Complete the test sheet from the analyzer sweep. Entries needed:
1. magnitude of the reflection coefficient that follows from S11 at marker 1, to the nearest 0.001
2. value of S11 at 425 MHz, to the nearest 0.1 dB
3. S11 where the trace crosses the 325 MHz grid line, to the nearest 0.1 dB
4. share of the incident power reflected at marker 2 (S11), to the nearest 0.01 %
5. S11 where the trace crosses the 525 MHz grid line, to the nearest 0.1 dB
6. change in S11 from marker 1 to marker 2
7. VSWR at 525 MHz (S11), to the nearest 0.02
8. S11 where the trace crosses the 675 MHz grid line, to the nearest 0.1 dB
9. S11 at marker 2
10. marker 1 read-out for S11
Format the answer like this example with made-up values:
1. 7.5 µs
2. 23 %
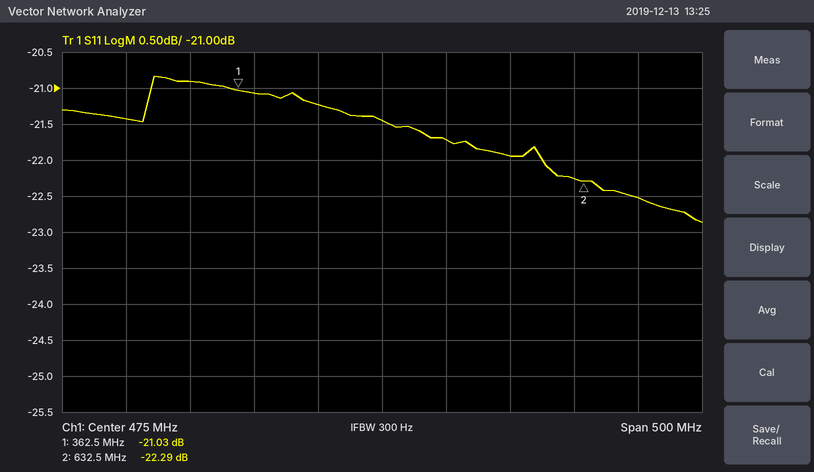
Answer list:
1. 0.089
2. -21.2 dB
3. -20.9 dB
4. 0.59 %
5. -21.7 dB
6. -1.26 dB
7. 1.18
8. -22.5 dB
9. -22.29 dB
10. -21.03 dB
